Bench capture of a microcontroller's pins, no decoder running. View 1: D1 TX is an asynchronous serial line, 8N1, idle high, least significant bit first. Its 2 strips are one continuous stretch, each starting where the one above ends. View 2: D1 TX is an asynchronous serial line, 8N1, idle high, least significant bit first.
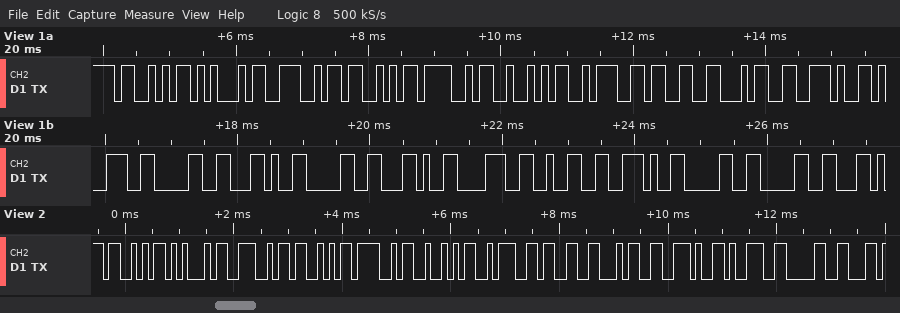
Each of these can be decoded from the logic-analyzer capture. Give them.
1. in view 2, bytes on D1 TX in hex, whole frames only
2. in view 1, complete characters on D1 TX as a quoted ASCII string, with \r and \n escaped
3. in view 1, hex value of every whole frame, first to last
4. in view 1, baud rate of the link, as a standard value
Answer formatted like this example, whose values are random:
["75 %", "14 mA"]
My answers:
["0x53 0x45 0x4E 0x53 0x4F 0x52 0x3A 0x33 0x34 0x2E 0x39 0x30", "\"SENSOR:34.90,0,82.00\"", "0x53 0x45 0x4E 0x53 0x4F 0x52 0x3A 0x33 0x34 0x2E 0x39 0x30 0x2C 0x30 0x2C 0x38 0x32 0x2E 0x30 0x30", "9600 baud"]
